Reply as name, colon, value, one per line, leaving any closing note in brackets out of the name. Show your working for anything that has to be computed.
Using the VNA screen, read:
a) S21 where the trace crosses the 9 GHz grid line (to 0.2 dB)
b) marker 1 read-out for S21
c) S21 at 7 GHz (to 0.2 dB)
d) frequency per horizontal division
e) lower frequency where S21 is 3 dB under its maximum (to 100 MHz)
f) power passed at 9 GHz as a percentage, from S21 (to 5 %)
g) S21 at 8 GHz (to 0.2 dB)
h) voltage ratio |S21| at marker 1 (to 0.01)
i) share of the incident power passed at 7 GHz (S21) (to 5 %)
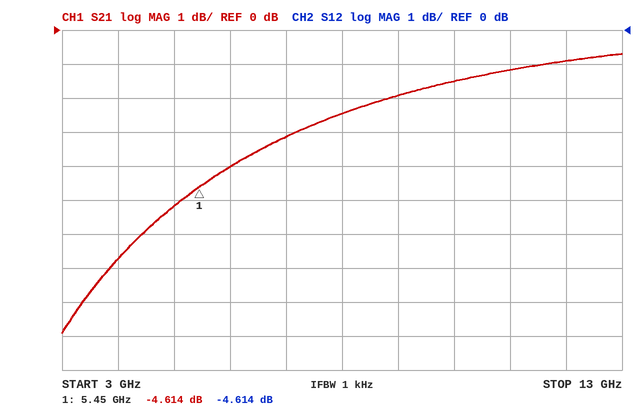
S21 where the trace crosses the 9 GHz grid line: -2.0 dB
marker 1 read-out for S21: -4.614 dB
S21 at 7 GHz: -3.2 dB
frequency per horizontal division: 1 GHz
lower frequency where S21 is 3 dB under its maximum: 6.3 GHz
power passed at 9 GHz as a percentage, from S21: 10^(-2/10) ≈ 63.1 %, so 65 % to the nearest 5 %
S21 at 8 GHz: -2.4 dB
voltage ratio |S21| at marker 1: 10^(-4.614/20) ≈ 0.59
share of the incident power passed at 7 GHz (S21): 10^(-3.2/10) ≈ 47.9 %, so 50 % to the nearest 5 %
